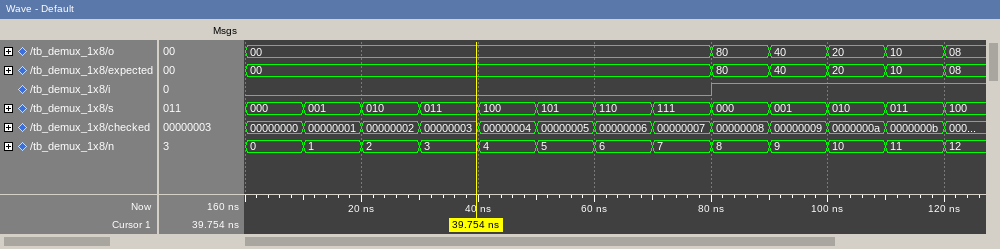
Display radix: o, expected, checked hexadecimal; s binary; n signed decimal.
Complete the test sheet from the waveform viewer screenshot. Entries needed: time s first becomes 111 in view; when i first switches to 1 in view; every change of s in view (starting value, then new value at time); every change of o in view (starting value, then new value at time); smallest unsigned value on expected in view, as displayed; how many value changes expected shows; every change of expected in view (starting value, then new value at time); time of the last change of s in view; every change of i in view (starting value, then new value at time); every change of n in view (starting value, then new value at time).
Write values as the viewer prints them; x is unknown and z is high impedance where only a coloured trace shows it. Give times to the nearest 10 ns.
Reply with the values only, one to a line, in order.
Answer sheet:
70 ns
80 ns
000, 001 at 10 ns, 010 at 20 ns, 011 at 30 ns, 100 at 40 ns, 101 at 50 ns, 110 at 60 ns, 111 at 70 ns, 000 at 80 ns, 001 at 90 ns, 010 at 100 ns, 011 at 110 ns, 100 at 120 ns
00, 80 at 80 ns, 40 at 90 ns, 20 at 100 ns, 10 at 110 ns, 08 at 120 ns
00
5
00, 80 at 80 ns, 40 at 90 ns, 20 at 100 ns, 10 at 110 ns, 08 at 120 ns
120 ns
0, 1 at 80 ns
0, 1 at 10 ns, 2 at 20 ns, 3 at 30 ns, 4 at 40 ns, 5 at 50 ns, 6 at 60 ns, 7 at 70 ns, 8 at 80 ns, 9 at 90 ns, 10 at 100 ns, 11 at 110 ns, 12 at 120 ns
